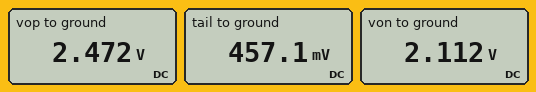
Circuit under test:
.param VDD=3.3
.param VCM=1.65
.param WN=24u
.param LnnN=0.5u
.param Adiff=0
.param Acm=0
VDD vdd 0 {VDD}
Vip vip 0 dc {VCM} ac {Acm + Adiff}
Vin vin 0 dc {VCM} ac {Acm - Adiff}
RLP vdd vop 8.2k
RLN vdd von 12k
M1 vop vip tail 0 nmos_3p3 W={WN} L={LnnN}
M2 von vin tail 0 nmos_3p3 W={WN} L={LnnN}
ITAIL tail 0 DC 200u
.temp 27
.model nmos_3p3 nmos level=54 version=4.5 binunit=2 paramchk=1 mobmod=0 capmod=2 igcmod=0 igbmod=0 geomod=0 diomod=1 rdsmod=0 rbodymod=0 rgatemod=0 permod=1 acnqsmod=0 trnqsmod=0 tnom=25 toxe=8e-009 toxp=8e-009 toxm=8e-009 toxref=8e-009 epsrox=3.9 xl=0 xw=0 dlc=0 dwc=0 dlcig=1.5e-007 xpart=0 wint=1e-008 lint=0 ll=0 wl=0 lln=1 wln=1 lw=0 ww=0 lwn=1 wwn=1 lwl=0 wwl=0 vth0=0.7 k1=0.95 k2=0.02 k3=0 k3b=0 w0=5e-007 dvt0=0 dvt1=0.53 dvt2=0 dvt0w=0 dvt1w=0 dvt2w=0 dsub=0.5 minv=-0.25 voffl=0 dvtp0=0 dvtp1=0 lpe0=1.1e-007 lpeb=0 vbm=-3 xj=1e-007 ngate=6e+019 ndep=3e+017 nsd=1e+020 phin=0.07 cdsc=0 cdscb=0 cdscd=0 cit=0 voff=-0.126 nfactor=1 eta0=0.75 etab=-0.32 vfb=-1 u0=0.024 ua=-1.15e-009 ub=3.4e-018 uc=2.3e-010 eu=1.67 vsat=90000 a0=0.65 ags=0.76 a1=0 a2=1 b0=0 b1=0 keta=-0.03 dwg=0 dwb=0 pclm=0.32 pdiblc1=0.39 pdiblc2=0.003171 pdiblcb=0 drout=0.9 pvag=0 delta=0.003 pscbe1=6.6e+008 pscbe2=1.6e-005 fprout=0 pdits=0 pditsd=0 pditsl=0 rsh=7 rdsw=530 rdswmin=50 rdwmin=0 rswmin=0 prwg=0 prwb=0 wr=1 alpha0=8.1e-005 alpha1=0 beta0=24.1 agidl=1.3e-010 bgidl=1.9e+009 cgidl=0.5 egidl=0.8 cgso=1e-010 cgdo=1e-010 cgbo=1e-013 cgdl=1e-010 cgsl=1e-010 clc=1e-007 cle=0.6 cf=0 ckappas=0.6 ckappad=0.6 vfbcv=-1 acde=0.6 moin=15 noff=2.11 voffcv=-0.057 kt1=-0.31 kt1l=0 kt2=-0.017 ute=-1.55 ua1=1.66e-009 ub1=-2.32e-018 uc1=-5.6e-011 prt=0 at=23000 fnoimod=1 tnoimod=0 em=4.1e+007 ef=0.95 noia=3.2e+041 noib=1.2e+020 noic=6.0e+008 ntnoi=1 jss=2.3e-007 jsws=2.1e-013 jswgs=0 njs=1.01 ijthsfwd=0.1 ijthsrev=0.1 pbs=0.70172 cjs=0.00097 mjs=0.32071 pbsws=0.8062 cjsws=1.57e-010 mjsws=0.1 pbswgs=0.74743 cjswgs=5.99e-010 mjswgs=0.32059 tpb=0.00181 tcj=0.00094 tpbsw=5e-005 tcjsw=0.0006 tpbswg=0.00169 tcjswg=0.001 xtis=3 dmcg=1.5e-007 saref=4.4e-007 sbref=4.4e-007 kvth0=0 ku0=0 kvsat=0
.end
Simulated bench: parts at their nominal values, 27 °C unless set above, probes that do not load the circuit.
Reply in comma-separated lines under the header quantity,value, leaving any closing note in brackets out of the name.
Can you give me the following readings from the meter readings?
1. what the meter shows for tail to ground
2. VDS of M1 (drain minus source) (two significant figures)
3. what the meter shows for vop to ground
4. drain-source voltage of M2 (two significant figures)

quantity,value
what the meter shows for tail to ground,457.1 mV
VDS of M1 (drain minus source),2.0 V
what the meter shows for vop to ground,2.472 V
drain-source voltage of M2,1.7 V
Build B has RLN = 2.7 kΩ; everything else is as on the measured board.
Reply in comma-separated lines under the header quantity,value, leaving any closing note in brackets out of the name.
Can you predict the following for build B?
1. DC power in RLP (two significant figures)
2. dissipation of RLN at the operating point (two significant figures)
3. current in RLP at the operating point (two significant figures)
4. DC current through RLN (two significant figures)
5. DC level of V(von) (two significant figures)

quantity,value
DC power in RLP,80 µW
dissipation of RLN at the operating point,29 µW
current in RLP at the operating point,99 µA
DC current through RLN,100 µA
DC level of V(von),3.0 V
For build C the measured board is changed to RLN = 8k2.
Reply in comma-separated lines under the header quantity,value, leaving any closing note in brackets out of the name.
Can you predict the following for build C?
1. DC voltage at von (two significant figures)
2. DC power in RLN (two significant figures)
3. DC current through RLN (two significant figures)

quantity,value
DC voltage at von,2.5 V
DC power in RLN,82 µW
DC current through RLN,100 µA
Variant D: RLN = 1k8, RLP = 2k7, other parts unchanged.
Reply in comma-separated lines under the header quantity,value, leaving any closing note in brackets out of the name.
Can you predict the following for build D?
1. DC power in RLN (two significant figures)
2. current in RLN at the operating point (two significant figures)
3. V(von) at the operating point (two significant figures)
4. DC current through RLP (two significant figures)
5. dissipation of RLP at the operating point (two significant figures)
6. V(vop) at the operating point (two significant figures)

quantity,value
DC power in RLN,19 µW
current in RLN at the operating point,100 µA
V(von) at the operating point,3.1 V
DC current through RLP,100 µA
dissipation of RLP at the operating point,28 µW
V(vop) at the operating point,3.0 V
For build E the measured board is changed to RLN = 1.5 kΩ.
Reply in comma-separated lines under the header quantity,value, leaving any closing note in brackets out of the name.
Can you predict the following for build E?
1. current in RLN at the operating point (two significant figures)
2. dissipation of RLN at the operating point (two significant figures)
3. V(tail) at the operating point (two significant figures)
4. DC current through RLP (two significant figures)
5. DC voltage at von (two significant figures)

quantity,value
current in RLN at the operating point,100 µA
dissipation of RLN at the operating point,16 µW
V(tail) at the operating point,460 mV
DC current through RLP,98 µA
DC voltage at von,3.1 V
